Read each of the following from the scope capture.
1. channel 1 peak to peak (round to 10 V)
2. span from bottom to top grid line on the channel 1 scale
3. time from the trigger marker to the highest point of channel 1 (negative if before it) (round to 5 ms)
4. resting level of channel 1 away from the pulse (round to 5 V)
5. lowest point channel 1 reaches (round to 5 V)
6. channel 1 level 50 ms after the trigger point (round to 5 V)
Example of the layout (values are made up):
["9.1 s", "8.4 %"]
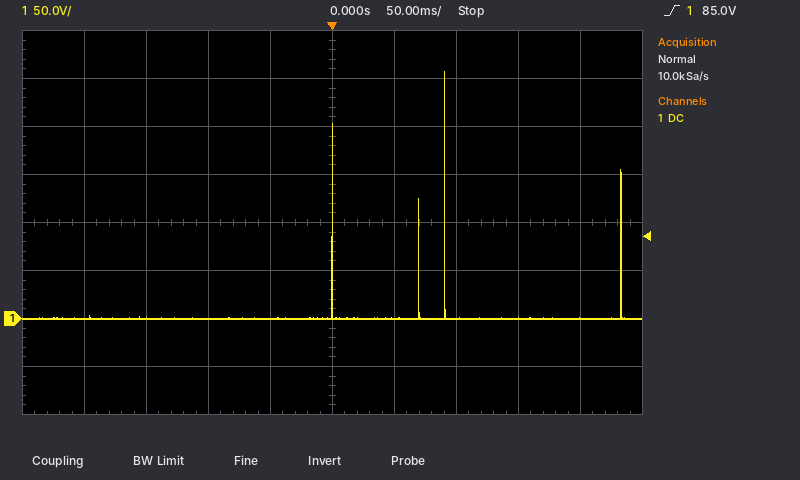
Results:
["260 V", "400 V", "+90 ms", "0 V", "0 V", "0 V"]
